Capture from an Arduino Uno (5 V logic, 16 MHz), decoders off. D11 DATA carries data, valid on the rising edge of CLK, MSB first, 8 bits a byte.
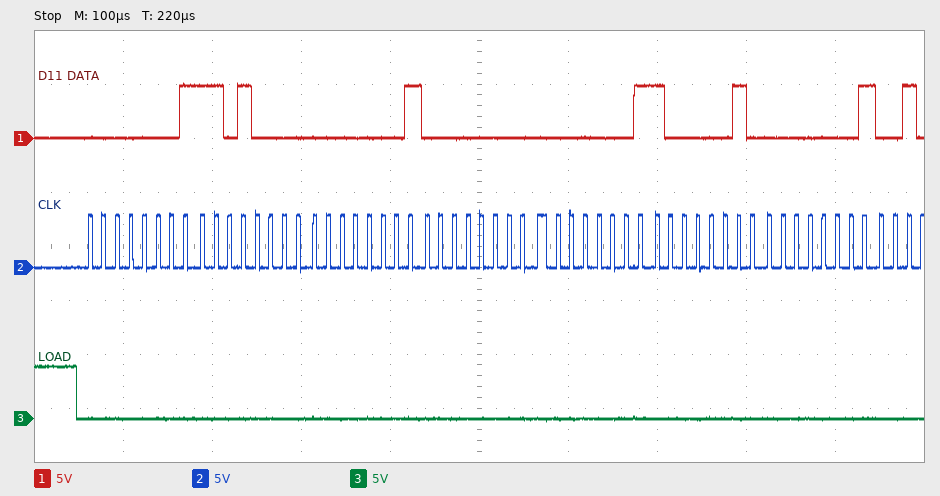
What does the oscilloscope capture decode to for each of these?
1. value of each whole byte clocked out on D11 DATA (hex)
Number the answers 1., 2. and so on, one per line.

1. 01 D0 01 00 01 82 01
